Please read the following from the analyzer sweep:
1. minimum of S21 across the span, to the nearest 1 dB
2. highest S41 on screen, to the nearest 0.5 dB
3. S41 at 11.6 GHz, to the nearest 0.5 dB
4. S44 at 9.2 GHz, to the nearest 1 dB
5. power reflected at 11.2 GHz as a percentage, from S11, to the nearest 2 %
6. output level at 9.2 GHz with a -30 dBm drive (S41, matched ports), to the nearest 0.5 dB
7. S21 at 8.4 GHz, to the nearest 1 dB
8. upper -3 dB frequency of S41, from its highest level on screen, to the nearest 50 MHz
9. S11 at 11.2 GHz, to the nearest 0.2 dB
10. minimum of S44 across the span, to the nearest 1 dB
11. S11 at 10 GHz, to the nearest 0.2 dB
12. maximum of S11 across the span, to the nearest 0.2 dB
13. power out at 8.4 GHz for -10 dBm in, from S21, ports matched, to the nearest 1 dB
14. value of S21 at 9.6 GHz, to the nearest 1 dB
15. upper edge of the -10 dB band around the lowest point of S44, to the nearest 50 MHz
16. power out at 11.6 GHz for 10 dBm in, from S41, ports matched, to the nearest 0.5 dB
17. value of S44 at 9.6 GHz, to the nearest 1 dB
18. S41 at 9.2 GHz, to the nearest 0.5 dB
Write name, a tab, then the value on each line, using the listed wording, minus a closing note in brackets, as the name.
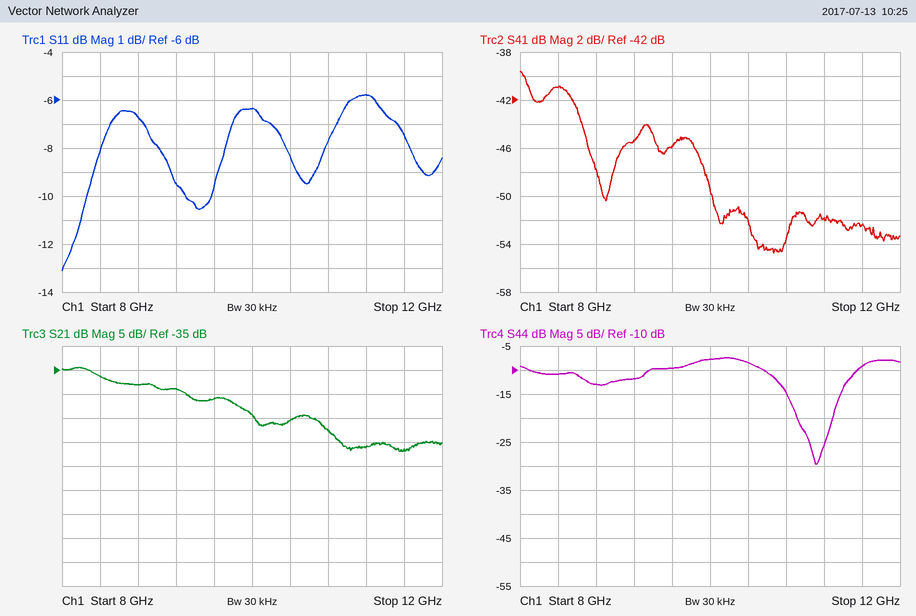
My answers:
minimum of S21 across the span, to the nearest 1 dB	-52 dB
highest S41 on screen, to the nearest 0.5 dB	-39.5 dB
S41 at 11.6 GHz, to the nearest 0.5 dB	-52.5 dB
S44 at 9.2 GHz, to the nearest 1 dB	-12 dB
power reflected at 11.2 GHz as a percentage, from S11, to the nearest 2 %	26 %
output level at 9.2 GHz with a -30 dBm drive (S41, matched ports), to the nearest 0.5 dB	-75.5 dBm
S21 at 8.4 GHz, to the nearest 1 dB	-36 dB
upper -3 dB frequency of S41, from its highest level on screen, to the nearest 50 MHz	8.60 GHz
S11 at 11.2 GHz, to the nearest 0.2 dB	-5.8 dB
minimum of S44 across the span, to the nearest 1 dB	-30 dB
S11 at 10 GHz, to the nearest 0.2 dB	-6.4 dB
maximum of S11 across the span, to the nearest 0.2 dB	-5.8 dB
power out at 8.4 GHz for -10 dBm in, from S21, ports matched, to the nearest 1 dB	-46 dBm
value of S21 at 9.6 GHz, to the nearest 1 dB	-41 dB
upper edge of the -10 dB band around the lowest point of S44, to the nearest 50 MHz	11.55 GHz
power out at 11.6 GHz for 10 dBm in, from S41, ports matched, to the nearest 0.5 dB	-42.5 dBm
value of S44 at 9.6 GHz, to the nearest 1 dB	-10 dB
S41 at 9.2 GHz, to the nearest 0.5 dB	-45.5 dB
